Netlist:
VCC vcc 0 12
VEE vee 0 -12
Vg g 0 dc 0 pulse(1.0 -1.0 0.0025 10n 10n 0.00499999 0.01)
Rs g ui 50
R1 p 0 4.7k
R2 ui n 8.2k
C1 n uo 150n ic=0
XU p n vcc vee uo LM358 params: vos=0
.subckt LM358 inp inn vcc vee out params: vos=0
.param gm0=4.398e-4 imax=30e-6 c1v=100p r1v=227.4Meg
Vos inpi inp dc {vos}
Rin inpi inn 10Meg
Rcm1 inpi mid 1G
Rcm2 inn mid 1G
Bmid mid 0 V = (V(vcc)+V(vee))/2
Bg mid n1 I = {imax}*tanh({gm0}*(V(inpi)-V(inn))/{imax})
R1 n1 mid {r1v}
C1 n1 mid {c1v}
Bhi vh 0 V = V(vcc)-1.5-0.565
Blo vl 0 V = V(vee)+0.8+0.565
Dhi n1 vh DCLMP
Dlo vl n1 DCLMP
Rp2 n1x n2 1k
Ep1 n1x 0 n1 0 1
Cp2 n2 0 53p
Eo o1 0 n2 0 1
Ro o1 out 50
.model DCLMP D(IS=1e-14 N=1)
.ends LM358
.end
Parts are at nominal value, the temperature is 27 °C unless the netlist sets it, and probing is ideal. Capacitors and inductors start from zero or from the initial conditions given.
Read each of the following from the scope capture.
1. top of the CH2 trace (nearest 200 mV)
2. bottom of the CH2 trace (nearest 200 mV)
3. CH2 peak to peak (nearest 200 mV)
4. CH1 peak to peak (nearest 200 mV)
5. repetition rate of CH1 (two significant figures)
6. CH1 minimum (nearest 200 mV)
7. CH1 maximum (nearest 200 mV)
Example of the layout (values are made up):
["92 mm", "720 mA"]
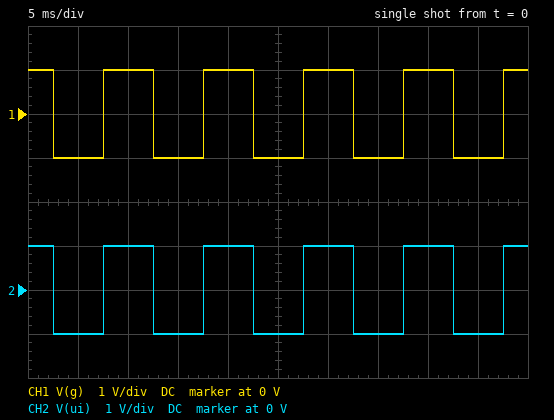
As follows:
["1.0 V", "-1.0 V", "2.0 V", "2.0 V", "100 Hz", "-1.0 V", "1.0 V"]
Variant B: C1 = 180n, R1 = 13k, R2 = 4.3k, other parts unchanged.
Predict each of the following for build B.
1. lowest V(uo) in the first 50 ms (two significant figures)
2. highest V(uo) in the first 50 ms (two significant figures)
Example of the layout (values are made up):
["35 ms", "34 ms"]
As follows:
["-3.2 V", "3.2 V"]
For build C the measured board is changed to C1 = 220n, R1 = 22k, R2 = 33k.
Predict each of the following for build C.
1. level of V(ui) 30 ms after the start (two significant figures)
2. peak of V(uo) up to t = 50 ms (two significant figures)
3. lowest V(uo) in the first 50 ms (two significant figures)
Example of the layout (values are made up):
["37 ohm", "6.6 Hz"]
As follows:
["1.0 V", "350 mV", "-350 mV"]
